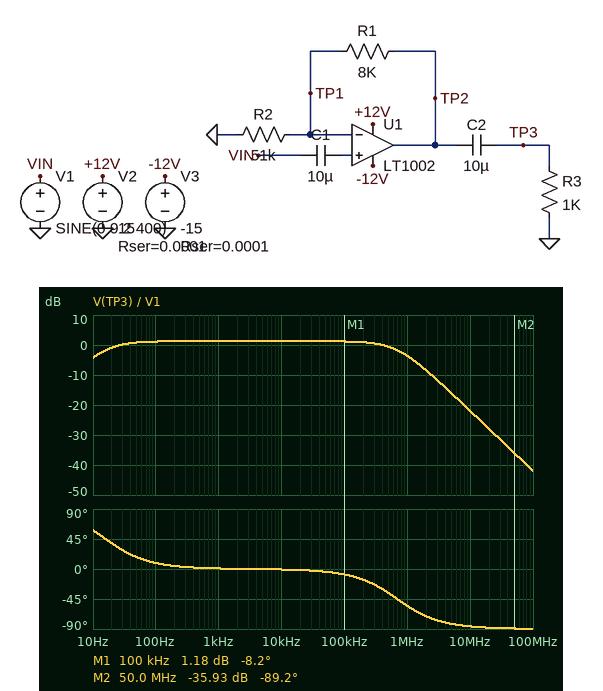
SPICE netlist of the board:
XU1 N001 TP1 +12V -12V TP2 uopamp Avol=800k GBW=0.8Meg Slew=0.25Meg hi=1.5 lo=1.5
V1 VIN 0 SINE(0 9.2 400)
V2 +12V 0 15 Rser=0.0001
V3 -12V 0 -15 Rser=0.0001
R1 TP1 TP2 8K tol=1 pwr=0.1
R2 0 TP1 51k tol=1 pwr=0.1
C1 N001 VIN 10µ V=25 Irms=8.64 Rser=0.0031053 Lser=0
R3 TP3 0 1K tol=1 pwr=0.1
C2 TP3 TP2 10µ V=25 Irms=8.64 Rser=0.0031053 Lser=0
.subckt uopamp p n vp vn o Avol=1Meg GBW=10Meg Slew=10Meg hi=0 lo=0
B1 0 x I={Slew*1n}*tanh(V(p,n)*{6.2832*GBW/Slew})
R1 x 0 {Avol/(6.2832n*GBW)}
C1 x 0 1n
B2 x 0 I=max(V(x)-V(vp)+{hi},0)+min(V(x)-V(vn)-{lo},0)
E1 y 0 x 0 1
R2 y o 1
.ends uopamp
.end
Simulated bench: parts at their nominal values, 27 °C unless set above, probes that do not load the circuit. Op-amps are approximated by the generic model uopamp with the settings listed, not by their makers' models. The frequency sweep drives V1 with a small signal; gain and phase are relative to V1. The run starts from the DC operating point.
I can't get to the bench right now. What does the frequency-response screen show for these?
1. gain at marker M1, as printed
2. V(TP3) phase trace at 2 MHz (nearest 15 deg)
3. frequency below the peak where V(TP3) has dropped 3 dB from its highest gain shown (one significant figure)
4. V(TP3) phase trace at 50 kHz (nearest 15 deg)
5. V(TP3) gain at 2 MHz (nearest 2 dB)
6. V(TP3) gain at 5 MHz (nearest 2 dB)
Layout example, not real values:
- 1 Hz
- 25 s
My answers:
- 1.18 dB
- -75 deg
- 20 Hz
- 0 deg
- -8 dB
- -16 dB
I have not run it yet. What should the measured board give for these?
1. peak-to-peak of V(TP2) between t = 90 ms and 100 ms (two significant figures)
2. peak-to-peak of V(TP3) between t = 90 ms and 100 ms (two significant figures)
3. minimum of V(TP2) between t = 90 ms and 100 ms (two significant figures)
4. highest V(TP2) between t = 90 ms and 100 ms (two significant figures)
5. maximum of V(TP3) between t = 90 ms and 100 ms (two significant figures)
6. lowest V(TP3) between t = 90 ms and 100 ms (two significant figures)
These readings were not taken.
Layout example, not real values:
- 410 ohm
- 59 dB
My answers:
- 21 V
- 21 V
- -11 V
- 11 V
- 11 V
- -11 V
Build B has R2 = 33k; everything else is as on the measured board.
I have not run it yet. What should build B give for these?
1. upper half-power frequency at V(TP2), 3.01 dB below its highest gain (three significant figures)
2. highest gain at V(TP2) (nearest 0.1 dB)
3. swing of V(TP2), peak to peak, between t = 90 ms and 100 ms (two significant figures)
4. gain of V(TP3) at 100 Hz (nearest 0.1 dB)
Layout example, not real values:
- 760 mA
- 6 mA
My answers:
- 643 kHz
- 1.9 dB
- 23 V
- 1.8 dB
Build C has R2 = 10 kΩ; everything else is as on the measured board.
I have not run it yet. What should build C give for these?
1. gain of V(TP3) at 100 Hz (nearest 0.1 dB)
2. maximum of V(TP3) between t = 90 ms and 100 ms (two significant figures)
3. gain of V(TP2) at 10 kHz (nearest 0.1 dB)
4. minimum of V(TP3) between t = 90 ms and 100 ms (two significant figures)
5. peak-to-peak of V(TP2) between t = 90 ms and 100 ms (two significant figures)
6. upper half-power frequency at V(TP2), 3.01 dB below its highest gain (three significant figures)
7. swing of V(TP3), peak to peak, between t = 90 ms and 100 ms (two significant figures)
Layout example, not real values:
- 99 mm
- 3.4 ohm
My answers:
- 5.0 dB
- 14 V
- 5.1 dB
- -14 V
- 27 V
- 444 kHz
- 28 V
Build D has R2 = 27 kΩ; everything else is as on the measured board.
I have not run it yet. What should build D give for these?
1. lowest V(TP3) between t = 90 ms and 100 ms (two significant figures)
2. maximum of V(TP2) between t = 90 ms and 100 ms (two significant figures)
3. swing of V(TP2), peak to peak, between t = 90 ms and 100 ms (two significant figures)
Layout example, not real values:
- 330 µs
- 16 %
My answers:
- -12 V
- 12 V
- 24 V
